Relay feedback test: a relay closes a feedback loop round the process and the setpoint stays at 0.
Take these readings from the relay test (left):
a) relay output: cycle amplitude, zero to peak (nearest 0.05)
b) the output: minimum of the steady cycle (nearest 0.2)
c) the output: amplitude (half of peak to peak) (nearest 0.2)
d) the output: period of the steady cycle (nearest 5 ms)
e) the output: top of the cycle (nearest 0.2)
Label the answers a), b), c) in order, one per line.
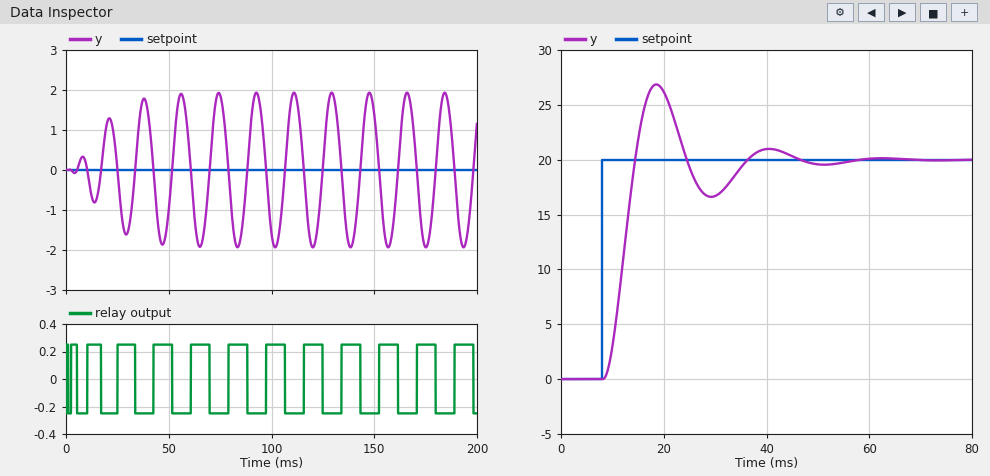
a) 0.25
b) -2.0
c) 2.0
d) 20 ms
e) 2.0
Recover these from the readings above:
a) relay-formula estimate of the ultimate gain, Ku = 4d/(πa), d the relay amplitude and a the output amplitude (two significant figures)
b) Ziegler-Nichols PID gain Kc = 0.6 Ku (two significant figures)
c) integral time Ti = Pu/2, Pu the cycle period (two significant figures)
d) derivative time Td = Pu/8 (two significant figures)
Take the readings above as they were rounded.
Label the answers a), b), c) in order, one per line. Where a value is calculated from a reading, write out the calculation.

a) 4 × 0.25 / (π × 2) = 0.16
b) 0.6 × 0.16 = 0.096
c) 20 / 2 = 10 ms
d) 20 / 8 = 2.5 ms
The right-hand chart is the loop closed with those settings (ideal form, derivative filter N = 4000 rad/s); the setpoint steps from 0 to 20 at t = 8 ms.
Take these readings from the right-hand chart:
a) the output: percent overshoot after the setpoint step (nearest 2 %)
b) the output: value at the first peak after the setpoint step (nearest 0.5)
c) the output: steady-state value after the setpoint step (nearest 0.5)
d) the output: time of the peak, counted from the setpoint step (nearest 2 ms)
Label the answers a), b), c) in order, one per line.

a) 34 %
b) 27.0
c) 20.0
d) 10 ms
